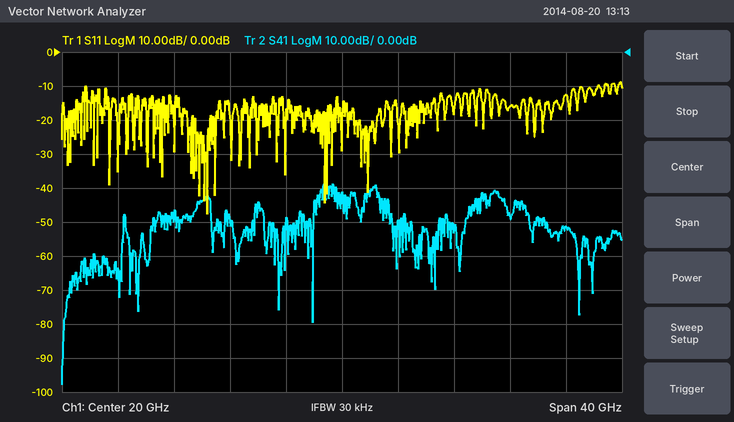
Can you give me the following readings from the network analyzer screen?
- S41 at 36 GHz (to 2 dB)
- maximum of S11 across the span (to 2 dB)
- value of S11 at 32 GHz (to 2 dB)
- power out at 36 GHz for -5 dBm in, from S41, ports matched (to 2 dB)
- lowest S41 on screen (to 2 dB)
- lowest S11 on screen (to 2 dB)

-52 dB
-8 dB
-16 dB
-56 dBm
-98 dB
-48 dB
